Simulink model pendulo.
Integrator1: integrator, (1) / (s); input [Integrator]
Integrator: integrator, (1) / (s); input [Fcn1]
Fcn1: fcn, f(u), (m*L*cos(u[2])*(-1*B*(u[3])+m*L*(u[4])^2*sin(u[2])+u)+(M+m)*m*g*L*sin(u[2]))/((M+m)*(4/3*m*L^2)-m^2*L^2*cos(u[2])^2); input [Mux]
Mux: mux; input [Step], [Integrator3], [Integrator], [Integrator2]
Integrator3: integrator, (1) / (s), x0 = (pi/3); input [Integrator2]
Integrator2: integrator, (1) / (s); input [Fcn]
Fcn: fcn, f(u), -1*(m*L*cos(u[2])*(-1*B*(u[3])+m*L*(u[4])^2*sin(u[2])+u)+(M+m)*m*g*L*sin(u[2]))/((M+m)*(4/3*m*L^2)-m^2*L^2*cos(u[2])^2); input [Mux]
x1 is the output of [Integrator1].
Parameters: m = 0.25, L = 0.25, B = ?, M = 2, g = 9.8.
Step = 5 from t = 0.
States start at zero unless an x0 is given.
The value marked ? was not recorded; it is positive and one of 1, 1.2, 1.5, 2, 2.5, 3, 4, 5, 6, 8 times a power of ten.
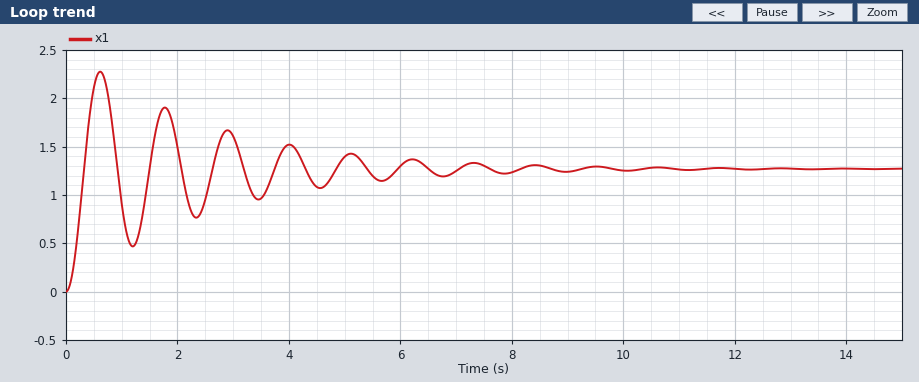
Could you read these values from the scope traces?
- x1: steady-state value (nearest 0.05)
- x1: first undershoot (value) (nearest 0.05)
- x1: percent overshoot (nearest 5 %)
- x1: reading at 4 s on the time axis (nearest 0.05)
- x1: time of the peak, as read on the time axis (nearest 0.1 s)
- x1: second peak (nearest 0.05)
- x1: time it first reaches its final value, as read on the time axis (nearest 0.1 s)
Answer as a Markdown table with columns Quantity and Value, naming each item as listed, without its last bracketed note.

| Quantity | Value |
|---|---|
| x1: steady-state value | 1.25 |
| x1: first undershoot (value) | 0.45 |
| x1: percent overshoot | 80 % |
| x1: reading at 4 s on the time axis | 1.50 |
| x1: time of the peak, as read on the time axis | 0.6 s |
| x1: second peak | 1.90 |
| x1: time it first reaches its final value, as read on the time axis | 0.3 s |
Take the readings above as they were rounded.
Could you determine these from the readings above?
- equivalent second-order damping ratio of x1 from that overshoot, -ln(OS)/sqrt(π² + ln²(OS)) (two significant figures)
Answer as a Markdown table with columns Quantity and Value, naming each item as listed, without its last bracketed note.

| Quantity | Value |
|---|---|
| equivalent second-order damping ratio of x1 from that overshoot, -ln(OS)/sqrt(π² + ln²(OS)) | 0.071 |
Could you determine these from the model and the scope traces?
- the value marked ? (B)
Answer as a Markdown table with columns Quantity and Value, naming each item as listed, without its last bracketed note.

| Quantity | Value |
|---|---|
| the value marked ? | 0.6 |
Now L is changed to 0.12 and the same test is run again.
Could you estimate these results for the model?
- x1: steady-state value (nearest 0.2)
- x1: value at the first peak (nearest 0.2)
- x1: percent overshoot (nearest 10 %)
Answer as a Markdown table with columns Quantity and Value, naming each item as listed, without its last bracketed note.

| Quantity | Value |
|---|---|
| x1: steady-state value | 1.2 |
| x1: value at the first peak | 2.2 |
| x1: percent overshoot | 70 % |
